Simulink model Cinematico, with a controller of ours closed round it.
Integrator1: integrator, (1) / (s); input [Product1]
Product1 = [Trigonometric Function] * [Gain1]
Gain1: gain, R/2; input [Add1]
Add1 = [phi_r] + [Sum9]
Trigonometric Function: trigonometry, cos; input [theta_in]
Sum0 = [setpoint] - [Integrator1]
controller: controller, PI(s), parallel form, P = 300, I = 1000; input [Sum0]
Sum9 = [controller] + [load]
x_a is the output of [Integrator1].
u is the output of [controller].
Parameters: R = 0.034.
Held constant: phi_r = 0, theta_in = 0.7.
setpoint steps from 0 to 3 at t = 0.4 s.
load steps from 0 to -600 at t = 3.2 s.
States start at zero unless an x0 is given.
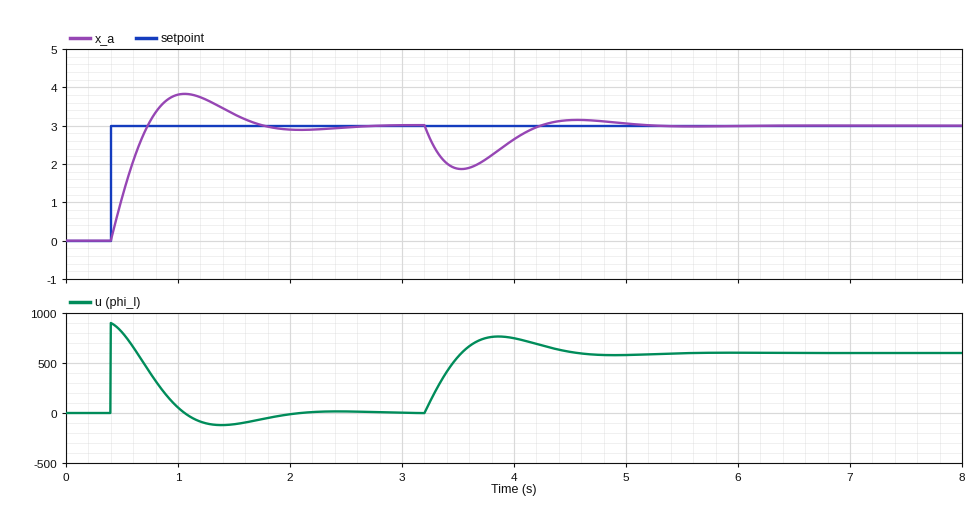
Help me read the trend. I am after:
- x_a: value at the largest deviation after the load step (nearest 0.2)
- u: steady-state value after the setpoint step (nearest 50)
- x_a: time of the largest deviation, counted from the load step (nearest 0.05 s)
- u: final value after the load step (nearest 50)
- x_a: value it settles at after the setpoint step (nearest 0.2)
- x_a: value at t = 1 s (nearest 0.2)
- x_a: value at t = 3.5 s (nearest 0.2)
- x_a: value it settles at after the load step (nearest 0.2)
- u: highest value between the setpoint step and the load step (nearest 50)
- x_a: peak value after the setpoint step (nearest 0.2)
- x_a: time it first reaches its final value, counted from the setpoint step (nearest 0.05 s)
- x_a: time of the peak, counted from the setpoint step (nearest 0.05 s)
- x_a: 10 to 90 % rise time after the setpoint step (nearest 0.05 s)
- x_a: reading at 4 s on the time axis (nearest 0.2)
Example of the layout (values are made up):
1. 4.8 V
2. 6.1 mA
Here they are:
1. 1.8
2. 0
3. 0.35 s
4. 600
5. 3.0
6. 3.8
7. 1.8
8. 3.0
9. 900
10. 3.8
11. 0.35 s
12. 0.65 s
13. 0.25 s
14. 2.6
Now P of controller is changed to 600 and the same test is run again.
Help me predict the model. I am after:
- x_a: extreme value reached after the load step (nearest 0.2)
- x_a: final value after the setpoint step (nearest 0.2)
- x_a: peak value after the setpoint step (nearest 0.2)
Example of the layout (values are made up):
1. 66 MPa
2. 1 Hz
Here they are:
1. 2.2
2. 3.0
3. 3.4
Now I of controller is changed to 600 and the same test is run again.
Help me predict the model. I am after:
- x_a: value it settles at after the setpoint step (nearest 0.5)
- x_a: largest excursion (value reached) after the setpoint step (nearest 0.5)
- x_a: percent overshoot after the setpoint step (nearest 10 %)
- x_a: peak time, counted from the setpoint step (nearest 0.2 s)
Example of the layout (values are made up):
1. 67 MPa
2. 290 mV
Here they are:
1. 3.0
2. 3.5
3. 20 %
4. 0.8 s
